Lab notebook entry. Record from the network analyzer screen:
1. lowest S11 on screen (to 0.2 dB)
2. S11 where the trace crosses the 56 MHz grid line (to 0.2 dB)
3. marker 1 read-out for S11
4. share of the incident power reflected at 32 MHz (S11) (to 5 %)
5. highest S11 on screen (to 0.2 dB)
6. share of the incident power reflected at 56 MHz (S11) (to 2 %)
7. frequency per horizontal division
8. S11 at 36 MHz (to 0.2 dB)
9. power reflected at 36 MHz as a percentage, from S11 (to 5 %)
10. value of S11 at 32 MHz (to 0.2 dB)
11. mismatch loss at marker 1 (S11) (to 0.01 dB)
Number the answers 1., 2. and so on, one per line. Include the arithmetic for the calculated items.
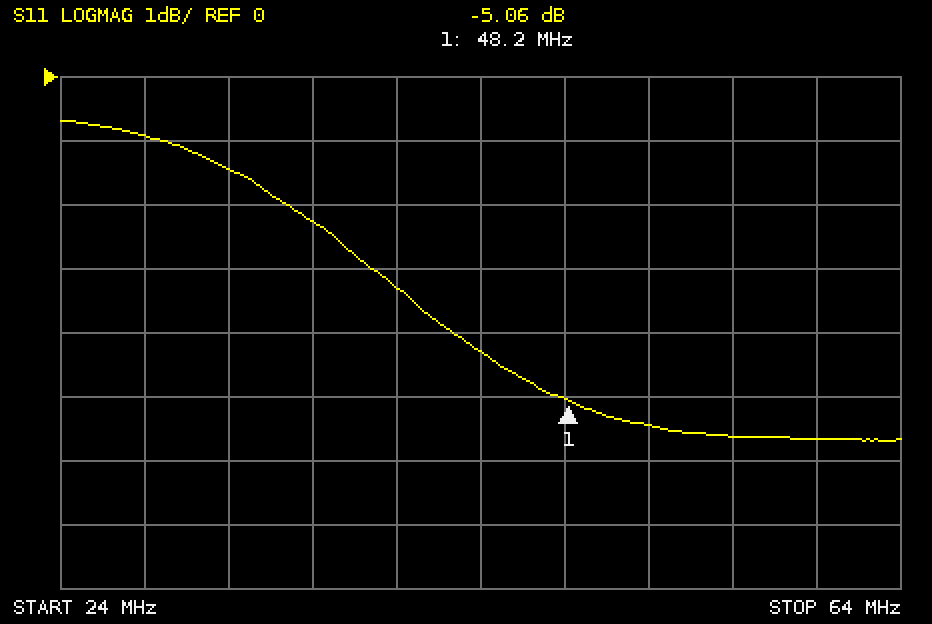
1. -5.6 dB
2. -5.6 dB
3. -5.06 dB
4. 10^(-1.4/10) ≈ 72.4 %, so 70 % to the nearest 5 %
5. -0.6 dB
6. 10^(-5.6/10) ≈ 28 %
7. 4 MHz
8. -2.2 dB
9. 10^(-2.2/10) ≈ 60 %
10. -1.4 dB
11. −10 log10(1 − 10^(-5.06/10)) ≈ 1.62 dB
